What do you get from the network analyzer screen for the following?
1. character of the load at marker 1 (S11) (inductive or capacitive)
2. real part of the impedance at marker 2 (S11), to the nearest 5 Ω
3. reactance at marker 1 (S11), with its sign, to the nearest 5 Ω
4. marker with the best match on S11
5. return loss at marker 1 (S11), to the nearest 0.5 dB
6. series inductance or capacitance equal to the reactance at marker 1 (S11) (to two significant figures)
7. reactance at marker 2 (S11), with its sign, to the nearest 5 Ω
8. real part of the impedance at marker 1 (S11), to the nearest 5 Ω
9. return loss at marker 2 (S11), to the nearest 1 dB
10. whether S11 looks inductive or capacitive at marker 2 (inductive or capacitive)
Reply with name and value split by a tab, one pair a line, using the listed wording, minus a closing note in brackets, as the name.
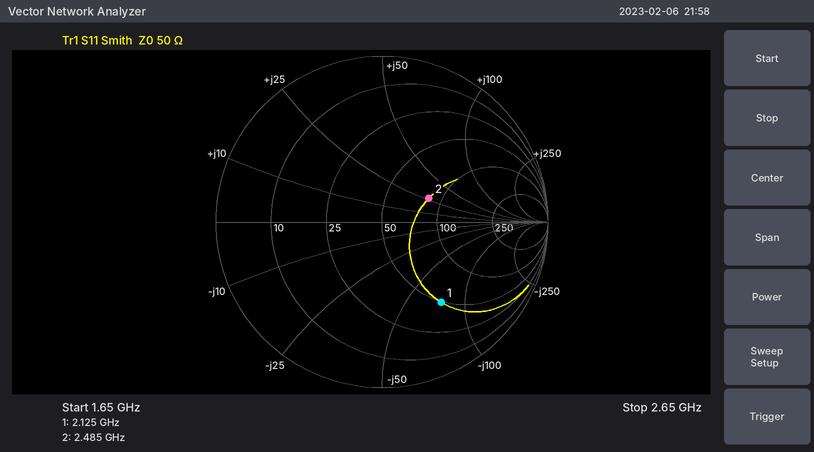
character of the load at marker 1 (S11)	capacitive
real part of the impedance at marker 2 (S11), to the nearest 5 Ω	85 Ω
reactance at marker 1 (S11), with its sign, to the nearest 5 Ω	-75 Ω
marker with the best match on S11	marker 2
return loss at marker 1 (S11), to the nearest 0.5 dB	4.5 dB
series inductance or capacitance equal to the reactance at marker 1 (S11)	1.0 pF
reactance at marker 2 (S11), with its sign, to the nearest 5 Ω	+25 Ω
real part of the impedance at marker 1 (S11), to the nearest 5 Ω	50 Ω
return loss at marker 2 (S11), to the nearest 1 dB	10 dB
whether S11 looks inductive or capacitive at marker 2	inductive
